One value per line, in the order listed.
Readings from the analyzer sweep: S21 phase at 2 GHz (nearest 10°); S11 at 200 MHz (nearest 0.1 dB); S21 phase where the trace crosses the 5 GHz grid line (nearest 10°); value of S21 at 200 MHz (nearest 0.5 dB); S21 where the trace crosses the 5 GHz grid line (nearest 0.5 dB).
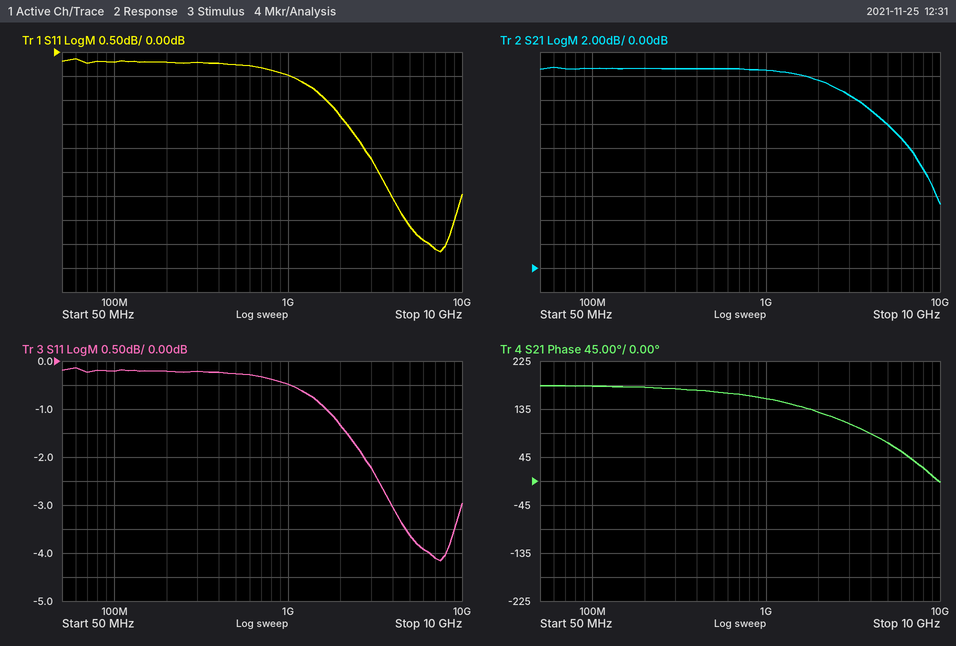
130°
-0.2 dB
70°
16.5 dB
12.0 dB
